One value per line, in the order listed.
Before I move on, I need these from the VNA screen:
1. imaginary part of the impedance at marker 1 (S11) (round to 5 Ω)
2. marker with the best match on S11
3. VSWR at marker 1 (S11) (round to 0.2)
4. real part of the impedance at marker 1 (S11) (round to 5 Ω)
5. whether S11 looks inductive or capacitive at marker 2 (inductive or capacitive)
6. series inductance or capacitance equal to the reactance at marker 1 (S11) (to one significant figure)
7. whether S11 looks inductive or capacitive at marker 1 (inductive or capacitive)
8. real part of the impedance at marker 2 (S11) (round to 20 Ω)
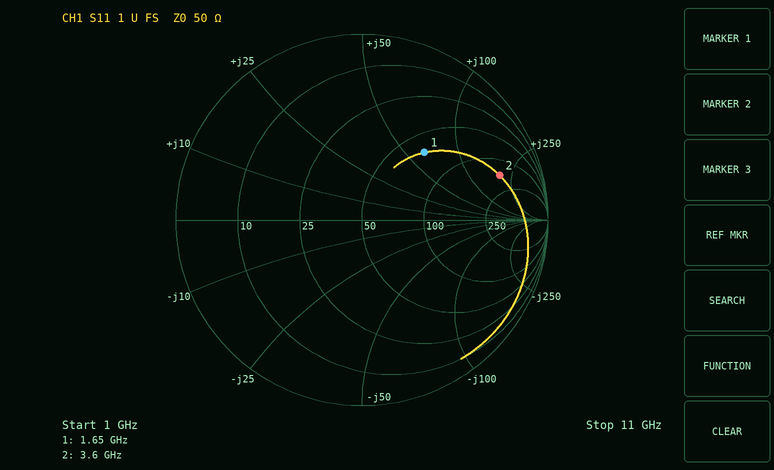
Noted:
+65 Ω
marker 1
3.0
65 Ω
inductive
6 nH
inductive
160 Ω
